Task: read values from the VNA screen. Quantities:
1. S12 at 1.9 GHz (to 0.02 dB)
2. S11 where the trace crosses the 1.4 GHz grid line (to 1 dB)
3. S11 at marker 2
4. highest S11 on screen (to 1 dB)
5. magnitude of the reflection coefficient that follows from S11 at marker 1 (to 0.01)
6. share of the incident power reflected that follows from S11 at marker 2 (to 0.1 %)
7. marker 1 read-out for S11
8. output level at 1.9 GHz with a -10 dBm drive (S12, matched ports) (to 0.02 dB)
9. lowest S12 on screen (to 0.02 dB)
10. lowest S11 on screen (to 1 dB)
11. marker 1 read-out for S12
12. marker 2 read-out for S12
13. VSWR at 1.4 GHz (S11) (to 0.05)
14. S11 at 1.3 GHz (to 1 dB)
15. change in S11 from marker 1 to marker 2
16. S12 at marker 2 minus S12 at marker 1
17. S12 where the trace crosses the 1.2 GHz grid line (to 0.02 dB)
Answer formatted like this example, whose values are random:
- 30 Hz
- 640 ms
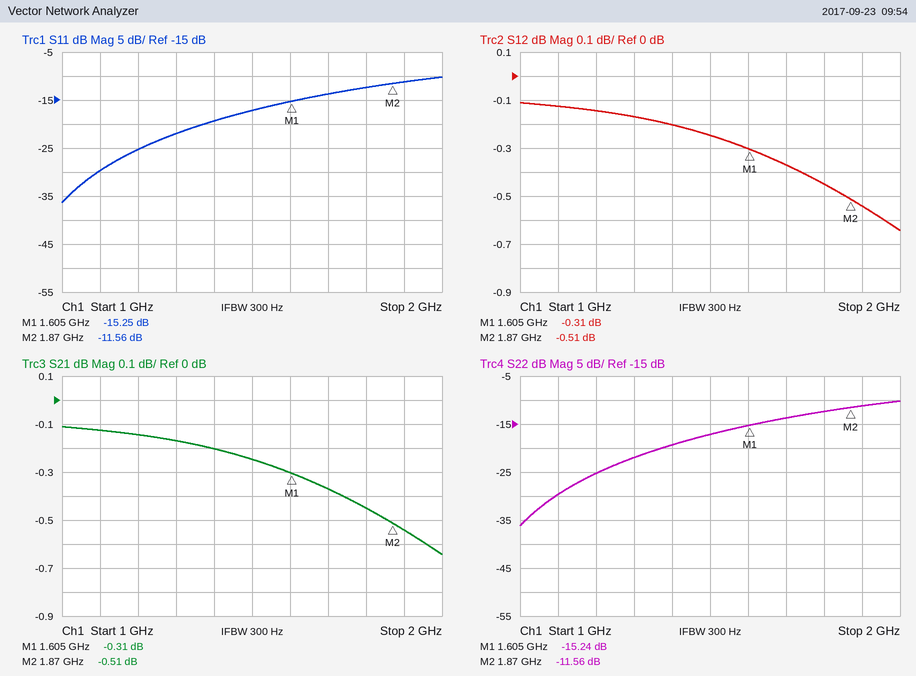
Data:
- -0.54 dB
- -19 dB
- -11.56 dB
- -10 dB
- 0.17
- 7.0 %
- -15.25 dB
- -10.54 dBm
- -0.64 dB
- -36 dB
- -0.31 dB
- -0.51 dB
- 1.25
- -22 dB
- 3.69 dB
- -0.20 dB
- -0.14 dB
